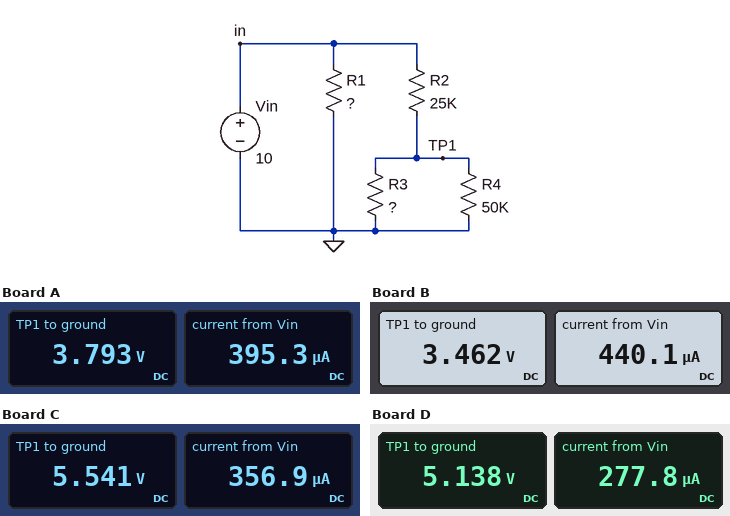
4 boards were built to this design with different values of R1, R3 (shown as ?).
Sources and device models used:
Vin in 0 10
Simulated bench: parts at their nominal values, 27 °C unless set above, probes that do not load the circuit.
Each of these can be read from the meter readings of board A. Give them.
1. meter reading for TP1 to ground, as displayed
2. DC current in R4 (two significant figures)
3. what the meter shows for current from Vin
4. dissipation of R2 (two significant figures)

3.793 V
76 µA
395.3 µA
1.5 mW
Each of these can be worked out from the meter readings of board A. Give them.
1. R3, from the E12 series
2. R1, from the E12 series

22 kΩ
68 kΩ
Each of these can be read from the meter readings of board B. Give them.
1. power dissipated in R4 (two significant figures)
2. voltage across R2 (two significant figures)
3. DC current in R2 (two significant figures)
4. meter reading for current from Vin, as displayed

240 µW
6.5 V
260 µA
440.1 µA
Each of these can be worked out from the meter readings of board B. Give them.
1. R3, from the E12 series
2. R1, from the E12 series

18 kΩ
56 kΩ
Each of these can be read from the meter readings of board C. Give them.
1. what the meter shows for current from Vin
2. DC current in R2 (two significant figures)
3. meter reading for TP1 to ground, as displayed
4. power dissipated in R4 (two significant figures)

356.9 µA
180 µA
5.541 V
610 µW
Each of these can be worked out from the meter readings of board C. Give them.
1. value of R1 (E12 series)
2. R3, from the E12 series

56 kΩ
82 kΩ
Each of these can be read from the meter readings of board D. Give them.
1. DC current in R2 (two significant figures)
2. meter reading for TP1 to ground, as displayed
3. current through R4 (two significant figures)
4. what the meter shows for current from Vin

190 µA
5.138 V
100 µA
277.8 µA
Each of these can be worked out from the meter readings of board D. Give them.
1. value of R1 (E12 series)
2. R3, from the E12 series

120 kΩ
56 kΩ
